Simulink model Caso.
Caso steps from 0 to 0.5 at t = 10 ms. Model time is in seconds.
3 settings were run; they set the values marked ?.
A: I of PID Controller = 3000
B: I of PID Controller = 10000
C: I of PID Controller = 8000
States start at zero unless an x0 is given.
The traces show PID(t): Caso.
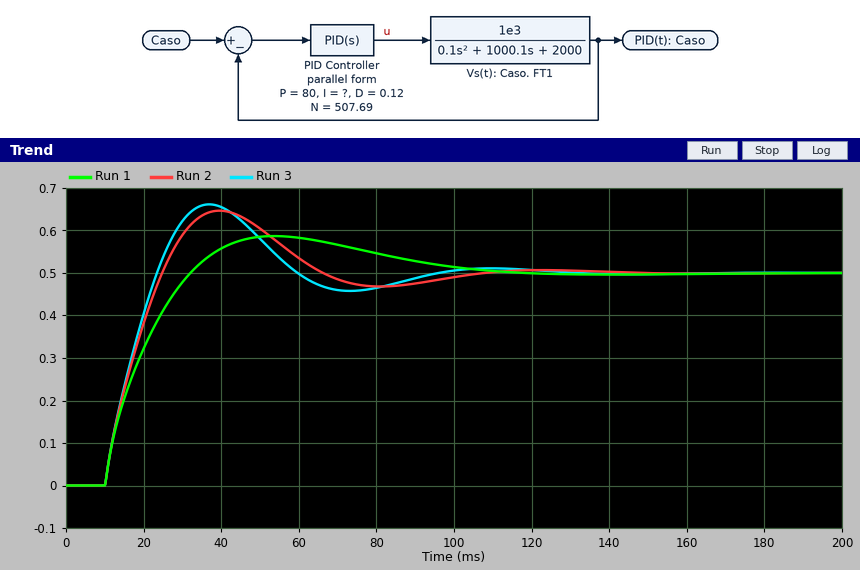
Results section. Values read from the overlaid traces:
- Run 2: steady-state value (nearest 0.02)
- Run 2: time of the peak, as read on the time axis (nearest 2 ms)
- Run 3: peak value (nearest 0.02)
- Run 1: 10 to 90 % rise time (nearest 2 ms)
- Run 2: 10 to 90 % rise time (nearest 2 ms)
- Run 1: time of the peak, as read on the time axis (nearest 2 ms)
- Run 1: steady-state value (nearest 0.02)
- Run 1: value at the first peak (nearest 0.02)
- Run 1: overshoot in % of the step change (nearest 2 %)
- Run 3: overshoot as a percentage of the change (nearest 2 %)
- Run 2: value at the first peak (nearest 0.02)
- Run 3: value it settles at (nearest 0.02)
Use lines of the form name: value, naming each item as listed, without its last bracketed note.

Run 2: steady-state value: 0.50
Run 2: time of the peak, as read on the time axis: 40 ms
Run 3: peak value: 0.66
Run 1: 10 to 90 % rise time: 16 ms
Run 2: 10 to 90 % rise time: 12 ms
Run 1: time of the peak, as read on the time axis: 54 ms
Run 1: steady-state value: 0.50
Run 1: value at the first peak: 0.58
Run 1: overshoot in % of the step change: 18 %
Run 3: overshoot as a percentage of the change: 32 %
Run 2: value at the first peak: 0.64
Run 3: value it settles at: 0.50
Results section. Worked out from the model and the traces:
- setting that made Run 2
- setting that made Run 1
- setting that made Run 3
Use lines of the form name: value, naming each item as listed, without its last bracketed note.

setting that made Run 2: C
setting that made Run 1: A
setting that made Run 3: B
